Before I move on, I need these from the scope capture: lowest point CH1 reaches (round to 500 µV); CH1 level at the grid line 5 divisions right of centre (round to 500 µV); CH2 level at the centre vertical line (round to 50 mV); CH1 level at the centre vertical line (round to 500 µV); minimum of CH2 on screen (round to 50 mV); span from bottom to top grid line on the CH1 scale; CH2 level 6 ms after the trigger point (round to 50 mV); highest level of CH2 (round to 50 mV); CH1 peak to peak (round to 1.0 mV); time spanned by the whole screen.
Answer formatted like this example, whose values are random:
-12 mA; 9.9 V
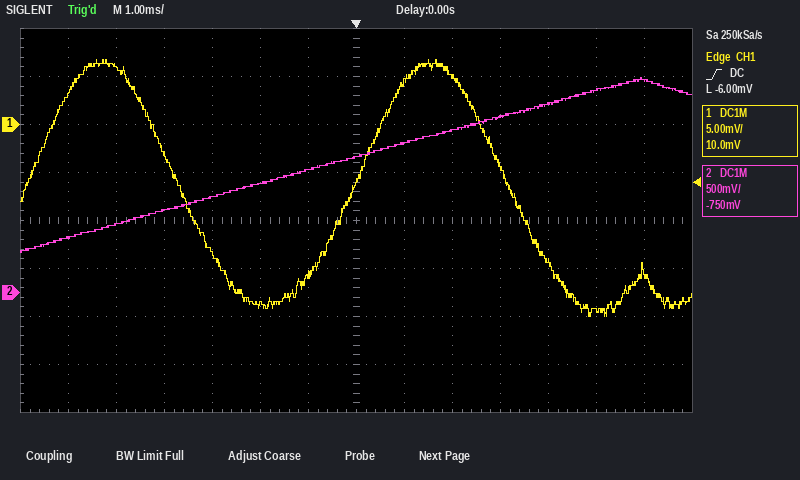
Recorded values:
-20.0 mV; -19.5 mV; 1.40 V; -6.0 mV; 400 mV; 40 mV; 2.20 V; 2.25 V; 27.0 mV; 14 ms
